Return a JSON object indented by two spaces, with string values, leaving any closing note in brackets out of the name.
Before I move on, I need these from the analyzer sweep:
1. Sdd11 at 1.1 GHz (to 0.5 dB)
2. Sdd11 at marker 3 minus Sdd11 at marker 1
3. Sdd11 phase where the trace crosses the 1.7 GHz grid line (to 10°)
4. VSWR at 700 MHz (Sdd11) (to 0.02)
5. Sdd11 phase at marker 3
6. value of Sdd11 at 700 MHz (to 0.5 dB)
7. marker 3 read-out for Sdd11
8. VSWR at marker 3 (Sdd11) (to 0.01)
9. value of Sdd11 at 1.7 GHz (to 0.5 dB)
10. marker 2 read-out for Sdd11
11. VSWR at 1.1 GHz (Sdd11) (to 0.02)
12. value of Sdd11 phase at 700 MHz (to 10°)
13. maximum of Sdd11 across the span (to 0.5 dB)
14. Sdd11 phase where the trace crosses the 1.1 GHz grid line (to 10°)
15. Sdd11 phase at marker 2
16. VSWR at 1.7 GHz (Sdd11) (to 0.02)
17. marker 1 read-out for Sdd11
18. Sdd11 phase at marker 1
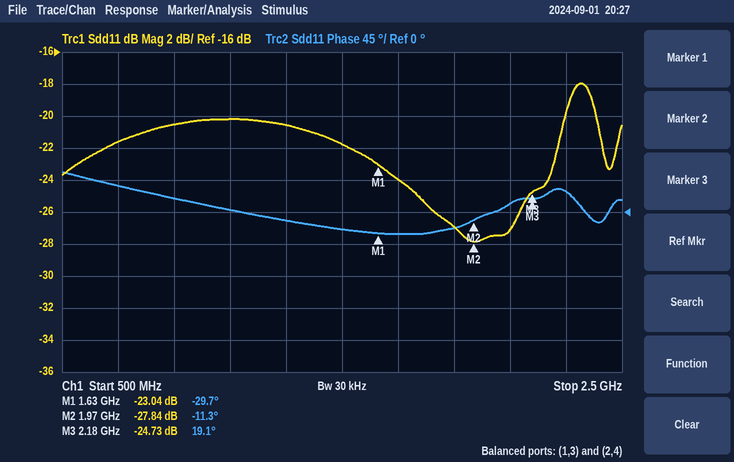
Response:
{
  "Sdd11 at 1.1 GHz": "-20.0 dB",
  "Sdd11 at marker 3 minus Sdd11 at marker 1": "-1.69 dB",
  "Sdd11 phase where the trace crosses the 1.7 GHz grid line": "-30°",
  "VSWR at 700 MHz (Sdd11)": "1.18",
  "Sdd11 phase at marker 3": "19.1°",
  "value of Sdd11 at 700 MHz": "-21.5 dB",
  "marker 3 read-out for Sdd11": "-24.73 dB",
  "VSWR at marker 3 (Sdd11)": "1.12",
  "value of Sdd11 at 1.7 GHz": "-24.0 dB",
  "marker 2 read-out for Sdd11": "-27.84 dB",
  "VSWR at 1.1 GHz (Sdd11)": "1.22",
  "value of Sdd11 phase at 700 MHz": "40°",
  "maximum of Sdd11 across the span": "-18.0 dB",
  "Sdd11 phase where the trace crosses the 1.1 GHz grid line": "0°",
  "Sdd11 phase at marker 2": "-11.3°",
  "VSWR at 1.7 GHz (Sdd11)": "1.14",
  "marker 1 read-out for Sdd11": "-23.04 dB",
  "Sdd11 phase at marker 1": "-29.7°"
}
